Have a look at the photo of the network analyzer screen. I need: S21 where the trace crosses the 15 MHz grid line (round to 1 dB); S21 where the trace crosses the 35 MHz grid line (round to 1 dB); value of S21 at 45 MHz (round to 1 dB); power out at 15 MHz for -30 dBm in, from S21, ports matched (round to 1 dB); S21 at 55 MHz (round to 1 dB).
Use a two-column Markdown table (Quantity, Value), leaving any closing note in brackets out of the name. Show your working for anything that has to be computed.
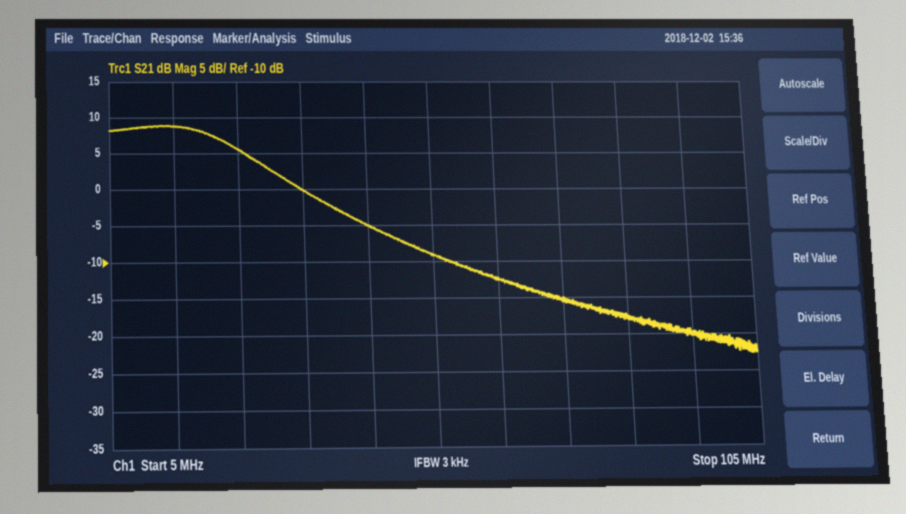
| Quantity | Value |
|---|---|
| S21 where the trace crosses the 15 MHz grid line | 9 dB |
| S21 where the trace crosses the 35 MHz grid line | 0 dB |
| value of S21 at 45 MHz | -5 dB |
| power out at 15 MHz for -30 dBm in, from S21, ports matched | -30 dBm + (9 dB) = -21 dBm |
| S21 at 55 MHz | -9 dB |
